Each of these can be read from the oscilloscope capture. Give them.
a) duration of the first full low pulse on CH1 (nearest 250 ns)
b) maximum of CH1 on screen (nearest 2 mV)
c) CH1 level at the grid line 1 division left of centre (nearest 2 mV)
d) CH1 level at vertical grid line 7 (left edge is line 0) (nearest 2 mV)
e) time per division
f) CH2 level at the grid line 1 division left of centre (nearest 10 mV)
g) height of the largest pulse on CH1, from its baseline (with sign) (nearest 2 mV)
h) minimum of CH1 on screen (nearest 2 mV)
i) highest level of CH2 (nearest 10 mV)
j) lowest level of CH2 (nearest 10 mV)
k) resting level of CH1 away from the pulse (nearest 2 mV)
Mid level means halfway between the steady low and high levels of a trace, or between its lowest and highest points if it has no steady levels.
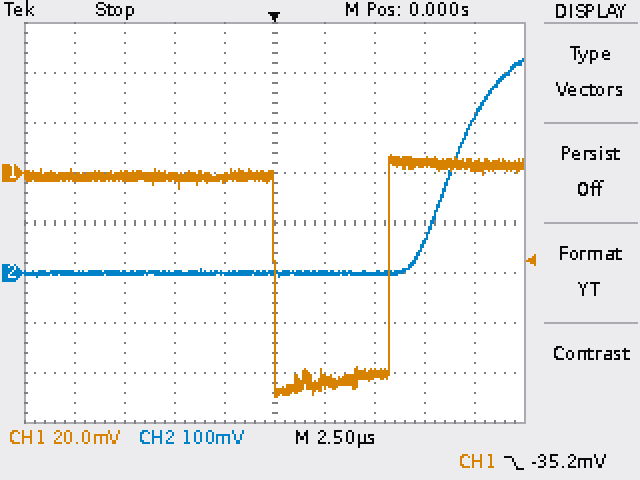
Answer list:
5.75 µs
8 mV
-2 mV
-80 mV
2.5 µs
0 mV
-88 mV
-90 mV
430 mV
-10 mV
-2 mV
